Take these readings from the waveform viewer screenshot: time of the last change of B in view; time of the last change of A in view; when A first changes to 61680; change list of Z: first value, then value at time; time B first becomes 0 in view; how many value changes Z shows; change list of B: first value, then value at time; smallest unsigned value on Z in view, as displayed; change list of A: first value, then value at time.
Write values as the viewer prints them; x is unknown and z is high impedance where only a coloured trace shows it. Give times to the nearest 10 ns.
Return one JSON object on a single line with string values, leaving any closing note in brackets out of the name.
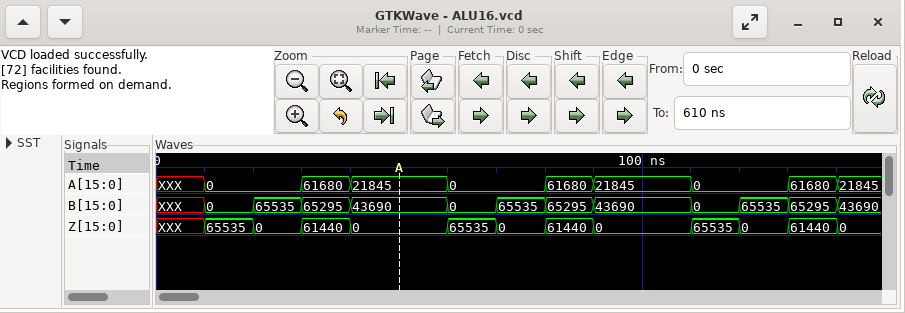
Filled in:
{"time of the last change of B in view": "140 ns", "time of the last change of A in view": "140 ns", "when A first changes to 61680": "30 ns", "change list of Z: first value, then value at time": "XXX, 65535 at 10 ns, 0 at 20 ns, 61440 at 30 ns, 0 at 40 ns, 65535 at 60 ns, 0 at 70 ns, 61440 at 80 ns, 0 at 90 ns, 65535 at 110 ns, 0 at 120 ns, 61440 at 130 ns, 0 at 140 ns", "time B first becomes 0 in view": "10 ns", "how many value changes Z shows": "12", "change list of B: first value, then value at time": "XXX, 0 at 10 ns, 65535 at 20 ns, 65295 at 30 ns, 43690 at 40 ns, 0 at 60 ns, 65535 at 70 ns, 65295 at 80 ns, 43690 at 90 ns, 0 at 110 ns, 65535 at 120 ns, 65295 at 130 ns, 43690 at 140 ns", "smallest unsigned value on Z in view, as displayed": "0", "change list of A: first value, then value at time": "XXX, 0 at 10 ns, 61680 at 30 ns, 21845 at 40 ns, 0 at 60 ns, 61680 at 80 ns, 21845 at 90 ns, 0 at 110 ns, 61680 at 130 ns, 21845 at 140 ns"}
